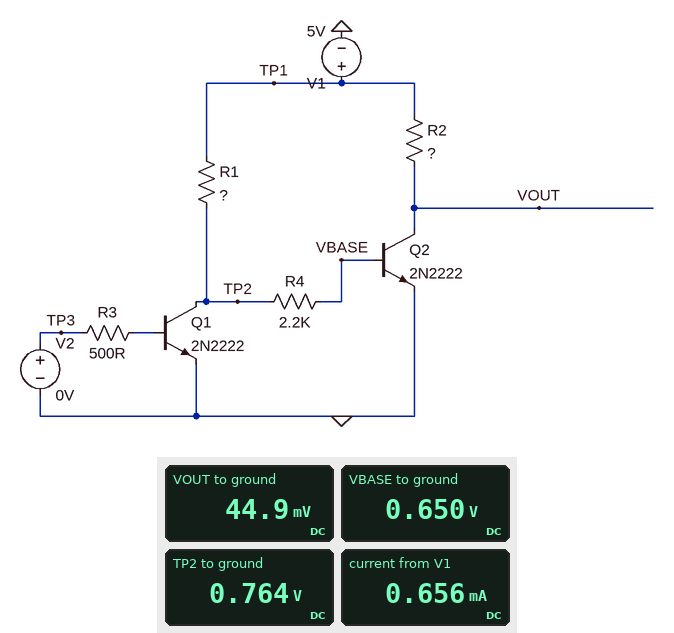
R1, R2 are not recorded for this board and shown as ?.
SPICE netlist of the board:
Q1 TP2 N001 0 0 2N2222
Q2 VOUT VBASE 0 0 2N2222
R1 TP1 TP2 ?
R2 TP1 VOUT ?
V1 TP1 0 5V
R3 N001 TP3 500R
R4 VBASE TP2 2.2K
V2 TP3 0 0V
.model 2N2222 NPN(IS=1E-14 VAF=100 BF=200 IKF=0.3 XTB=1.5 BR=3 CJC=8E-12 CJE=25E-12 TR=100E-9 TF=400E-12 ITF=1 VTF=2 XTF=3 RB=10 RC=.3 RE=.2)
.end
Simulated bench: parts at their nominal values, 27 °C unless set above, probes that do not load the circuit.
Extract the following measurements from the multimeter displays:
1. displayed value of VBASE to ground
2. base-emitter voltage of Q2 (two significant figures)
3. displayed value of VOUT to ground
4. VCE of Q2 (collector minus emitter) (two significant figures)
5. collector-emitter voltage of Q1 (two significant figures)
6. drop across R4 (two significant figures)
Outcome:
0.650 V
650 mV
44.9 mV
45 mV
760 mV
110 mV
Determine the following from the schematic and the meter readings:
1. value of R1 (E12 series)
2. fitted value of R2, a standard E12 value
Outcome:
82 kΩ
8.2 kΩ
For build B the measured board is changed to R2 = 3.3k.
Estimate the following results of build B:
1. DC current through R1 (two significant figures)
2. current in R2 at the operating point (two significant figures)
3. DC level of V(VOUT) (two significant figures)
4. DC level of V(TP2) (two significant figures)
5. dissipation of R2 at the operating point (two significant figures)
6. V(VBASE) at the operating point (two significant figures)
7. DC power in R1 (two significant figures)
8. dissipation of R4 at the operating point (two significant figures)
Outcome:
51 µA
1.5 mA
67 mV
780 mV
7.4 mW
670 mV
220 µW
5.8 µW
